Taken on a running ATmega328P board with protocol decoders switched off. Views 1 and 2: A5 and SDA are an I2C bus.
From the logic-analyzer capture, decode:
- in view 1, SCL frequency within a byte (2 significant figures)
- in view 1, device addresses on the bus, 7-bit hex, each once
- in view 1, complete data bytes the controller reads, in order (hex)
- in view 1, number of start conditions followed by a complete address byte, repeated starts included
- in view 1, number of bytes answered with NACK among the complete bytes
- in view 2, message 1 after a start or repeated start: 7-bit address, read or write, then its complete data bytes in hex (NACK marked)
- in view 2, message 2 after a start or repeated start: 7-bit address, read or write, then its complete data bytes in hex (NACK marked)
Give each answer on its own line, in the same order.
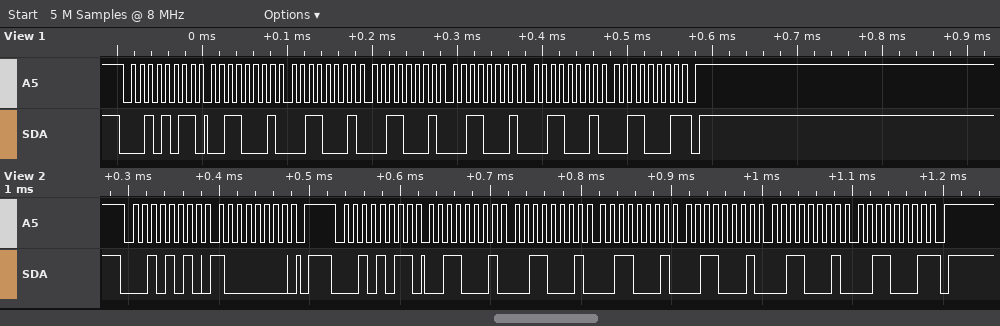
100 kHz
0x15
31 31 31 31 31 31
1
1
0x15 write: 80
0x15 read: 31 31 31 31 31 31 NACK
